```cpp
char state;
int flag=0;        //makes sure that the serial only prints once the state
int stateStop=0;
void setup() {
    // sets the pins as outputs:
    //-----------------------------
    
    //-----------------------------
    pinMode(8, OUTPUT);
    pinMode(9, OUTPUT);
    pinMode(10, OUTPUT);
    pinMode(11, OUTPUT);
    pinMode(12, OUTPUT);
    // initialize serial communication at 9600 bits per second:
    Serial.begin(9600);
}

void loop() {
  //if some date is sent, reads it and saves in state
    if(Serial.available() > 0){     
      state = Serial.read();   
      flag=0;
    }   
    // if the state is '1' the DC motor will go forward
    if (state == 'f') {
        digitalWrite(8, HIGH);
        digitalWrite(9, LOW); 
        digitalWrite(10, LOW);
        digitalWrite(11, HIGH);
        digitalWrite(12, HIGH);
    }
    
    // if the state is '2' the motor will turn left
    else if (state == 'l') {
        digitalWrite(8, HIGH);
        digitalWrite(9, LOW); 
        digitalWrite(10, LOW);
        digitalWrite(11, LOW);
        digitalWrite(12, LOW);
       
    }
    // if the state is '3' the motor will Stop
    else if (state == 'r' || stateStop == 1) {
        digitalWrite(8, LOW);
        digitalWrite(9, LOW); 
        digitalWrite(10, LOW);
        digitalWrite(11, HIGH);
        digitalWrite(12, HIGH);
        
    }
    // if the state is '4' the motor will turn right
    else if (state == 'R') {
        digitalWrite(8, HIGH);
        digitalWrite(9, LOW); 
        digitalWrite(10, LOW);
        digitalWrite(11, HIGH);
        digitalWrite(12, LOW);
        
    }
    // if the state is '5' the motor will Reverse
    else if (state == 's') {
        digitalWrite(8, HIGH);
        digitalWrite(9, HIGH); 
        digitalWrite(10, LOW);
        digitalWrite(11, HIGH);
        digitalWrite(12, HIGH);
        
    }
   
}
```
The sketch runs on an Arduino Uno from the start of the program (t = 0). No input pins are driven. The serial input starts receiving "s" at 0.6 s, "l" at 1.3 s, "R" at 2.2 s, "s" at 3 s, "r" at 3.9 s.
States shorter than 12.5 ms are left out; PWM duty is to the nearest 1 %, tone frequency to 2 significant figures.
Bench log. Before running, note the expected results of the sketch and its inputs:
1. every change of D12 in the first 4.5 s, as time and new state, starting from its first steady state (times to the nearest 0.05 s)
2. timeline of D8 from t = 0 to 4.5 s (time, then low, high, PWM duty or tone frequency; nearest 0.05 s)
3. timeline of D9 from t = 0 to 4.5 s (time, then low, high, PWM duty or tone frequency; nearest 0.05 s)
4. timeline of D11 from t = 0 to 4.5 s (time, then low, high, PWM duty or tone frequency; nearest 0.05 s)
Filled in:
0 s low; 0.6 s high; 1.3 s low; 3 s high
0 s low; 0.6 s high; 3.9 s low
0 s low; 0.6 s high; 1.3 s low; 3 s high; 3.9 s low
0 s low; 0.6 s high; 1.3 s low; 2.2 s high
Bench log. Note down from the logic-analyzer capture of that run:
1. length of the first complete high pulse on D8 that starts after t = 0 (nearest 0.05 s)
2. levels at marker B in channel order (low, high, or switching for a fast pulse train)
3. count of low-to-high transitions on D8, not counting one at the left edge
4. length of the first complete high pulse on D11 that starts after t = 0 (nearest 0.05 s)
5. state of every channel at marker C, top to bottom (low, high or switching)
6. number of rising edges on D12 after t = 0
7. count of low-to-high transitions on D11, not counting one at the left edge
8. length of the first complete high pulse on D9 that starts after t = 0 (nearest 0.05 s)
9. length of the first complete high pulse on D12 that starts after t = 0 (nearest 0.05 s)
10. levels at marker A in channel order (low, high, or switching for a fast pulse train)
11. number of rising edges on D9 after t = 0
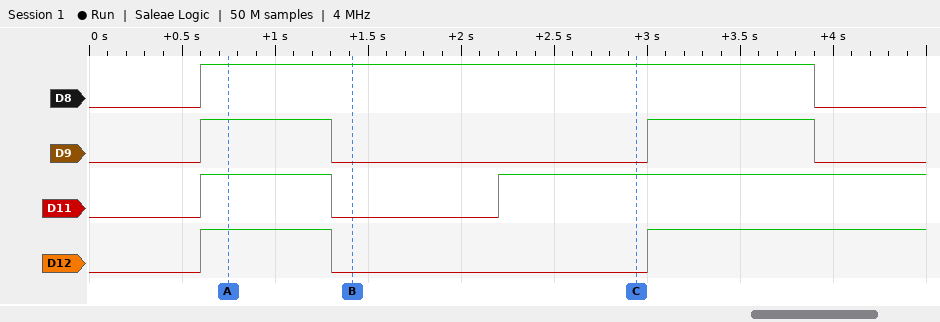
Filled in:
3.30 s
D8 high, D9 low, D11 low, D12 low
1
0.70 s
D8 high, D9 low, D11 high, D12 low
2
2
0.70 s
0.70 s
D8 high, D9 high, D11 high, D12 high
2
